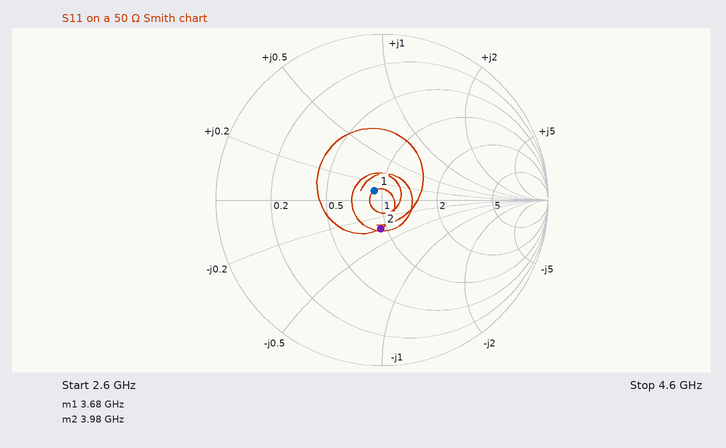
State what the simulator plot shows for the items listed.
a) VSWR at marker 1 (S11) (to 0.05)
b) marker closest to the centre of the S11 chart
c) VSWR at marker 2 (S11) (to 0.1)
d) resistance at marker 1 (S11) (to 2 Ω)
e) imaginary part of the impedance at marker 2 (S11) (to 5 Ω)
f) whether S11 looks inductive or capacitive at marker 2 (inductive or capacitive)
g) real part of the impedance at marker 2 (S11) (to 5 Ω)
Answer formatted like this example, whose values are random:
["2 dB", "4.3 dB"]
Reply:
["1.15", "marker 1", "1.4", "46 Ω", "-15 Ω", "capacitive", "45 Ω"]
